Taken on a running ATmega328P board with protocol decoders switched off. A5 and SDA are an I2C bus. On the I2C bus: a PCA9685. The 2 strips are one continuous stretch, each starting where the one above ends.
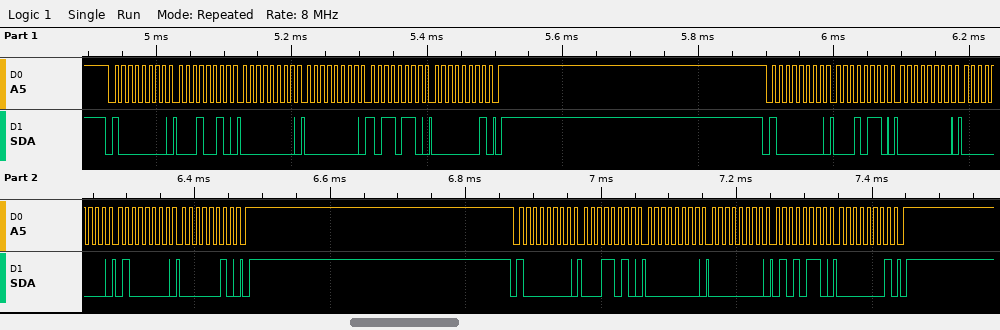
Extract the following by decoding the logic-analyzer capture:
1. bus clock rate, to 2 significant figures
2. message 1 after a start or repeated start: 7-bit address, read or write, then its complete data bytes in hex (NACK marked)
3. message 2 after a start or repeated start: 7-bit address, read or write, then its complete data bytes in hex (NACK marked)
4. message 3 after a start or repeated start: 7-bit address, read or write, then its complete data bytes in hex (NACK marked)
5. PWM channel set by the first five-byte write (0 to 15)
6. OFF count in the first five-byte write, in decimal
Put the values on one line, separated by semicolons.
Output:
100 kHz; 0x40 write: 12 00 00 B6 01; 0x40 write: 16 00 00 40 02; 0x40 write: 1A 00 00 56 01; 3; 438
